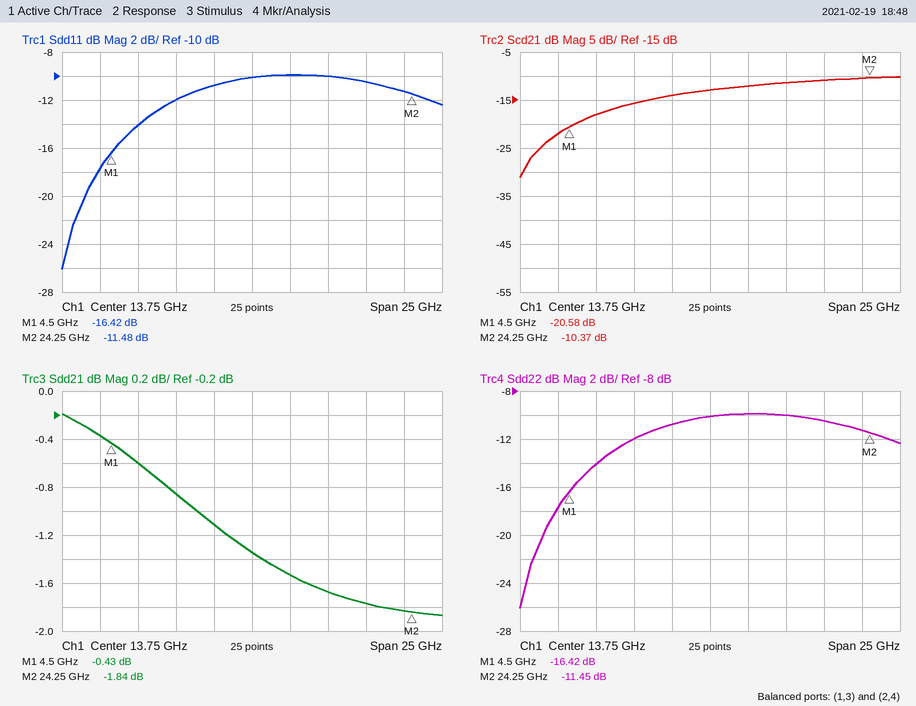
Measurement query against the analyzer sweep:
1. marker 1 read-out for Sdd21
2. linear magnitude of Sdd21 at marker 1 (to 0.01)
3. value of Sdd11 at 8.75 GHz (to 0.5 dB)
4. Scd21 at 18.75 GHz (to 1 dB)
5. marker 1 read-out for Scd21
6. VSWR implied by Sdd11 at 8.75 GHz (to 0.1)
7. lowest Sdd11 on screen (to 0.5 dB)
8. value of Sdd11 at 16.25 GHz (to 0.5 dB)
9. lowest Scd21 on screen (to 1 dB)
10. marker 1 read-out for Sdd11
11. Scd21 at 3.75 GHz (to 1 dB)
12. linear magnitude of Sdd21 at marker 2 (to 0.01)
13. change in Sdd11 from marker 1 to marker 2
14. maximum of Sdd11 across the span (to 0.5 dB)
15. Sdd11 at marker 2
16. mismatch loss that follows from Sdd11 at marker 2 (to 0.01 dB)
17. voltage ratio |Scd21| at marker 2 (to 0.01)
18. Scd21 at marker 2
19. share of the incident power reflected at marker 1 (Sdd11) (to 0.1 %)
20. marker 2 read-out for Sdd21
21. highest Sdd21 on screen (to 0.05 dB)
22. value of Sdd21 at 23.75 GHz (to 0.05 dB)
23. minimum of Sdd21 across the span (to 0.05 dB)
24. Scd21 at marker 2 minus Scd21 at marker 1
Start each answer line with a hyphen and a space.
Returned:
- -0.43 dB
- 0.95
- -12.0 dB
- -11 dB
- -20.58 dB
- 1.7
- -26.0 dB
- -10.0 dB
- -31 dB
- -16.42 dB
- -22 dB
- 0.81
- 4.94 dB
- -10.0 dB
- -11.48 dB
- 0.32 dB
- 0.30
- -10.37 dB
- 2.3 %
- -1.84 dB
- -0.20 dB
- -1.85 dB
- -1.85 dB
- 10.21 dB
